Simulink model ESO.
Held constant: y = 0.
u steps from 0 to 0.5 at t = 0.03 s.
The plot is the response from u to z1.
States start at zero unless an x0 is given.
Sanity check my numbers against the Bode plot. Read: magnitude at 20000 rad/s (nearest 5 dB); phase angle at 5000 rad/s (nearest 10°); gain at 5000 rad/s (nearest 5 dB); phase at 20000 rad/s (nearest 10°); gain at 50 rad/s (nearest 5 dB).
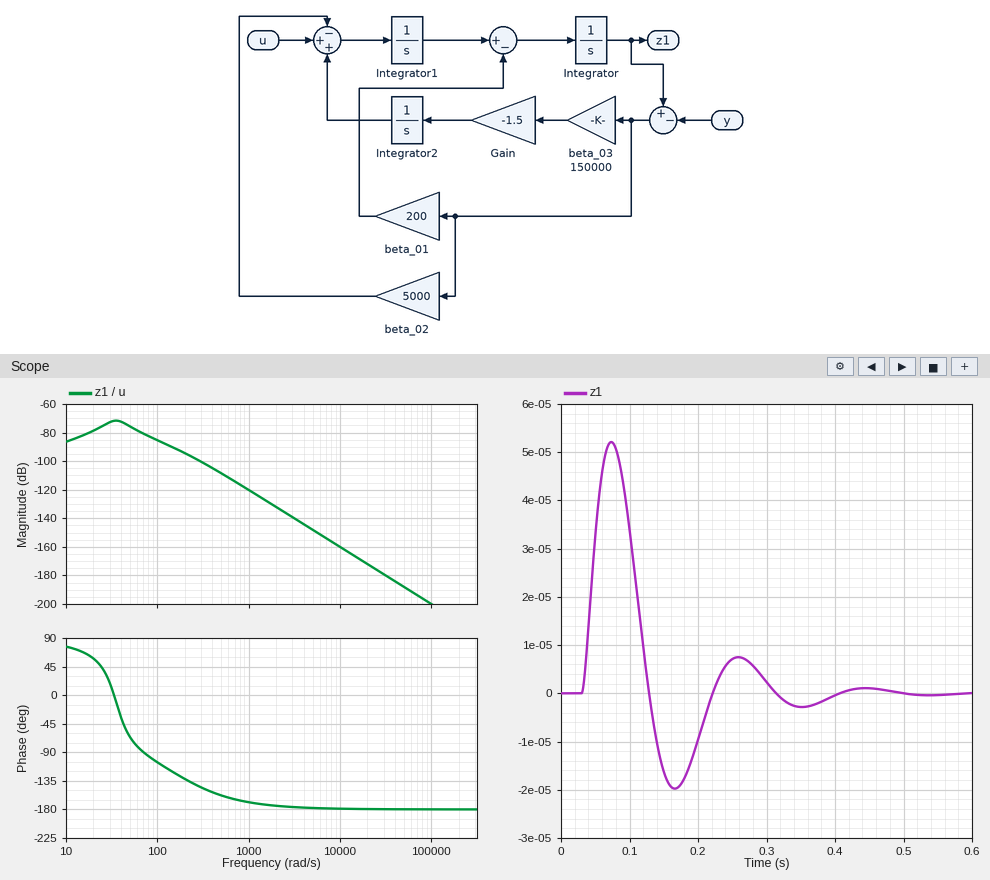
-170 dB
-180°
-150 dB
-180°
-75 dB
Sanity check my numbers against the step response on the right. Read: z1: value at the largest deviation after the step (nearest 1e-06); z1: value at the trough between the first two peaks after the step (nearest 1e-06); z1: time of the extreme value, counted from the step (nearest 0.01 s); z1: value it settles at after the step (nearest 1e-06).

0.000052
-0.000020
0.04 s
0.000000
